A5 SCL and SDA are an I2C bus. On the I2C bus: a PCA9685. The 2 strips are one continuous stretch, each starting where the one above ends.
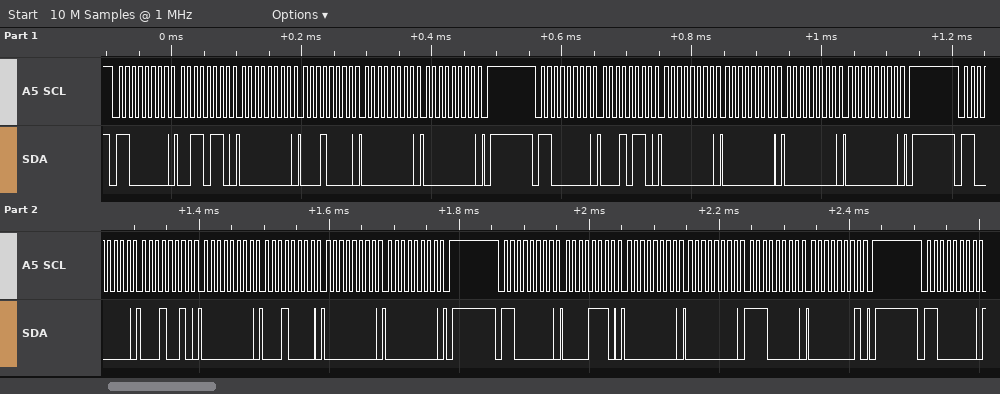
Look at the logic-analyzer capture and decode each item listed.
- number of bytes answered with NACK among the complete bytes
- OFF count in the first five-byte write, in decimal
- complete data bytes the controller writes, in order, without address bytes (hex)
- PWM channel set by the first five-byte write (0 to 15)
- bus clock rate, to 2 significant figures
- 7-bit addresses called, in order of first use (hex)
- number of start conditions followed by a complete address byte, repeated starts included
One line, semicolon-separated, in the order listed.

0; 0; 36 00 10 00 00 16 00 00 00 00 12 00 10 00 00 0E 00 00 E0 01; 12; 100 kHz; 0x60; 5
